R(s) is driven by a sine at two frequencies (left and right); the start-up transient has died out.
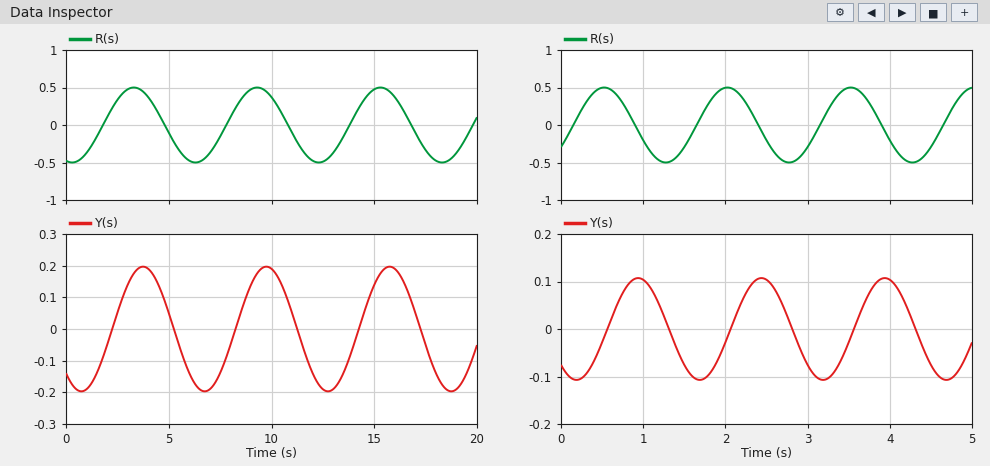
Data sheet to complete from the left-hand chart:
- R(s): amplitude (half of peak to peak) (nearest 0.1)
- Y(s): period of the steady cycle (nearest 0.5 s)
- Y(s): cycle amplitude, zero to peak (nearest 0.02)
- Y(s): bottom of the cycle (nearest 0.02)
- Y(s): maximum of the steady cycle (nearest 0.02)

0.5
6.0 s
0.20
-0.20
0.20
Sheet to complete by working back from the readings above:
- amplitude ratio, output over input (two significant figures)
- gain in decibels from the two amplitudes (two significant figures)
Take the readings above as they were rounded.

0.40
-8.0 dB
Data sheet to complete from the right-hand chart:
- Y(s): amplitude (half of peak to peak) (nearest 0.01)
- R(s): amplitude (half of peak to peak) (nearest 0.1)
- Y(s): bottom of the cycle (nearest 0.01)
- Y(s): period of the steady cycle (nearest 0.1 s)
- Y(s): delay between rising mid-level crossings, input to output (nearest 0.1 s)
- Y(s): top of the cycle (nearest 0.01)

0.11
0.5
-0.11
1.5 s
0.4 s
0.11
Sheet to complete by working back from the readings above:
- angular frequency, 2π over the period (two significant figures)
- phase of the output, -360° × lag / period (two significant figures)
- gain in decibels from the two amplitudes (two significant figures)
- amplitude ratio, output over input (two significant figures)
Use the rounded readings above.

4.2 rad/s
-96°
-13 dB
0.22
